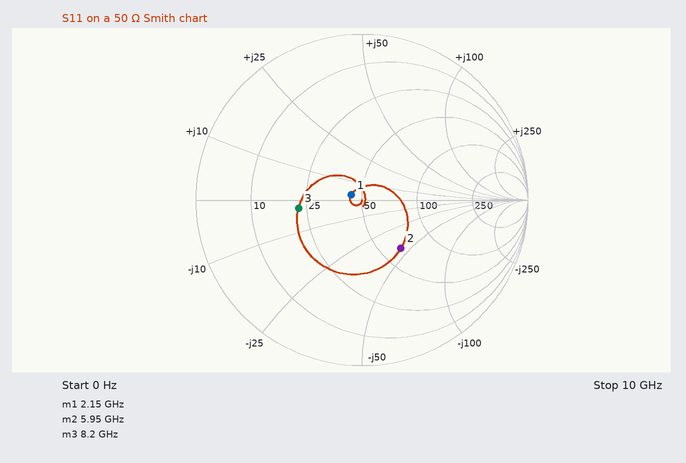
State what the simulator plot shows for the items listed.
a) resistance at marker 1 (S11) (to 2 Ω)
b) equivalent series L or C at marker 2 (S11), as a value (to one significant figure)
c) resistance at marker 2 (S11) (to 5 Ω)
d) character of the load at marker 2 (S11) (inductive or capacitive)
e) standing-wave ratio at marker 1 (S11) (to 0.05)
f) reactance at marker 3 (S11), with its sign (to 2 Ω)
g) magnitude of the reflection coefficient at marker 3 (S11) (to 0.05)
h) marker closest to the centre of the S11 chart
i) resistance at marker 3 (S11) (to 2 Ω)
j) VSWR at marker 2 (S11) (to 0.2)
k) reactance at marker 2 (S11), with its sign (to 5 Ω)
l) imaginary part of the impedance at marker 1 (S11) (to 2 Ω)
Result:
44 Ω
600 fF
65 Ω
capacitive
1.15
-2 Ω
0.40
marker 1
22 Ω
2.2
-45 Ω
+2 Ω
